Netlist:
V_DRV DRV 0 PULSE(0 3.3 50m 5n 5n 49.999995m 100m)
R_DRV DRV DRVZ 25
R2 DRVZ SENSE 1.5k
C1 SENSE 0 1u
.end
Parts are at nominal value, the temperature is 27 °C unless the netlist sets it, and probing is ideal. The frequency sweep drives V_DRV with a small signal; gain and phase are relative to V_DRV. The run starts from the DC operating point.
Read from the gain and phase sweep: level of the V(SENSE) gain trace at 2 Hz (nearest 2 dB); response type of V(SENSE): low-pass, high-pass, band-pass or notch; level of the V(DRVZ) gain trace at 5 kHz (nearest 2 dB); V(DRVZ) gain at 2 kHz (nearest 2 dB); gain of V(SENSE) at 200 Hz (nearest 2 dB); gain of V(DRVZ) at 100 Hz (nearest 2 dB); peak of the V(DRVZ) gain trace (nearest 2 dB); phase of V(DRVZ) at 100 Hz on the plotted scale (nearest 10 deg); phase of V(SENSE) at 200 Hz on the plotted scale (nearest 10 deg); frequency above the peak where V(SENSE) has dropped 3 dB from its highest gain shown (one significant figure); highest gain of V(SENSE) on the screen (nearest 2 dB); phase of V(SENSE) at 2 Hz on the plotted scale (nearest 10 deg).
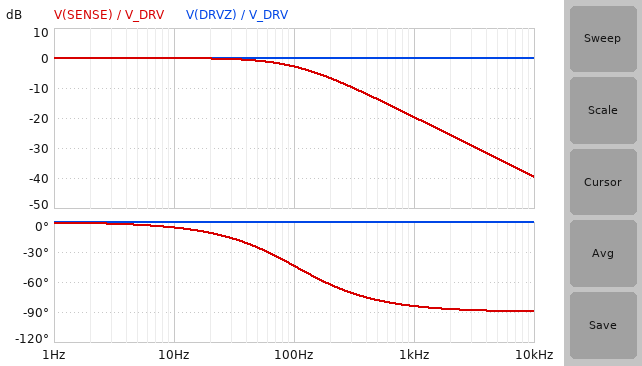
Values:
0 dB
low-pass
0 dB
0 dB
-6 dB
0 dB
0 dB
0 deg
-60 deg
100 Hz
0 dB
0 deg
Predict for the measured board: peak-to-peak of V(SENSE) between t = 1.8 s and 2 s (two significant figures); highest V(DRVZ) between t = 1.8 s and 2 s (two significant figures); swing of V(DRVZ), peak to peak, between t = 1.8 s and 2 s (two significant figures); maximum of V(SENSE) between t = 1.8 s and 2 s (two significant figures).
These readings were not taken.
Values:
3.3 V
3.3 V
3.3 V
3.3 V
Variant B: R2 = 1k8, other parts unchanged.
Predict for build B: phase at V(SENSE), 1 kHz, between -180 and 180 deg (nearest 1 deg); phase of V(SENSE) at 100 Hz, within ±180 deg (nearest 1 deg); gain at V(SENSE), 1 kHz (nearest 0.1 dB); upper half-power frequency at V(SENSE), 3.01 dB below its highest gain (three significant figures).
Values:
-85 deg
-49 deg
-21.2 dB
87.2 Hz
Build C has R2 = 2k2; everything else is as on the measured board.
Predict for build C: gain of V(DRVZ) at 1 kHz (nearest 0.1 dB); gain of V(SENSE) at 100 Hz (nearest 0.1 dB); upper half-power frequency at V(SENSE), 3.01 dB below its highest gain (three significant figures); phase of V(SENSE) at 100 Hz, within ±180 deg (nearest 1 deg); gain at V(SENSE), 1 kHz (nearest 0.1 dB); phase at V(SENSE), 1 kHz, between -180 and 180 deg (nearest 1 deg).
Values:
-0.1 dB
-4.7 dB
71.5 Hz
-54 deg
-22.9 dB
-86 deg
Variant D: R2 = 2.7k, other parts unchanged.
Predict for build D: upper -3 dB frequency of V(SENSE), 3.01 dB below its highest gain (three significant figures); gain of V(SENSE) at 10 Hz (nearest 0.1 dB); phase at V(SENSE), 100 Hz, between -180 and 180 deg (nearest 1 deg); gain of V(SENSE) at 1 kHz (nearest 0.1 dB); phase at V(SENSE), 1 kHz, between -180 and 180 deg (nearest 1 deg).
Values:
58.4 Hz
-0.1 dB
-60 deg
-24.7 dB
-87 deg
